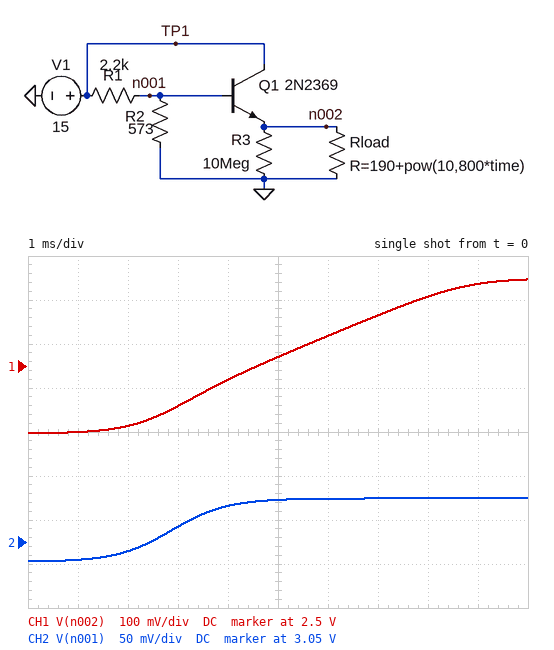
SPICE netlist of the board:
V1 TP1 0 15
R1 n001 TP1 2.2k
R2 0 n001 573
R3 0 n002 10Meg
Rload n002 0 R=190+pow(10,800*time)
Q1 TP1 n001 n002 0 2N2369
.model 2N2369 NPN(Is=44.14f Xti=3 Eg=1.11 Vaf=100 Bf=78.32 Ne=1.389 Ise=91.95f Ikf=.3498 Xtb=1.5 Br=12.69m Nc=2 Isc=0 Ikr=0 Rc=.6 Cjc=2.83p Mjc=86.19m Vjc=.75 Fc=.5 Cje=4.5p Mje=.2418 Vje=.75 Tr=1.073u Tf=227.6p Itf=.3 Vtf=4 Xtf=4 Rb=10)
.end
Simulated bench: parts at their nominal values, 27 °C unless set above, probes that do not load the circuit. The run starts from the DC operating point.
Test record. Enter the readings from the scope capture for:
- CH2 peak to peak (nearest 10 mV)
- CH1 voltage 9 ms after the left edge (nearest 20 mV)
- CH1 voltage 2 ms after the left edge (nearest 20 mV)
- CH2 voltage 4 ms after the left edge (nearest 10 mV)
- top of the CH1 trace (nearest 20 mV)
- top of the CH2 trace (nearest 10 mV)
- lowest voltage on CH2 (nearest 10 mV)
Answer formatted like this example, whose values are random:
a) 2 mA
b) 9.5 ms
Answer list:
a) 70 mV
b) 2.68 V
c) 2.36 V
d) 3.09 V
e) 2.70 V
f) 3.10 V
g) 3.03 V
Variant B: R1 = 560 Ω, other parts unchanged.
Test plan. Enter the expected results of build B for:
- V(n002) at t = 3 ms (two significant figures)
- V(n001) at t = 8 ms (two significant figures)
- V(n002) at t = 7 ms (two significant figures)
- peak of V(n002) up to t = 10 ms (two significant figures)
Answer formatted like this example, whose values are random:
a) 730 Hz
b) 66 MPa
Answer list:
a) 6.8 V
b) 7.6 V
c) 7.1 V
d) 7.2 V
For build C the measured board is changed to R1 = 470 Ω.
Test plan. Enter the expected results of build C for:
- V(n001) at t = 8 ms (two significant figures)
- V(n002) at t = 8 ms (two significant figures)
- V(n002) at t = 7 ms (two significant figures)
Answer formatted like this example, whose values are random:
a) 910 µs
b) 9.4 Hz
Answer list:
a) 8.2 V
b) 7.8 V
c) 7.7 V
